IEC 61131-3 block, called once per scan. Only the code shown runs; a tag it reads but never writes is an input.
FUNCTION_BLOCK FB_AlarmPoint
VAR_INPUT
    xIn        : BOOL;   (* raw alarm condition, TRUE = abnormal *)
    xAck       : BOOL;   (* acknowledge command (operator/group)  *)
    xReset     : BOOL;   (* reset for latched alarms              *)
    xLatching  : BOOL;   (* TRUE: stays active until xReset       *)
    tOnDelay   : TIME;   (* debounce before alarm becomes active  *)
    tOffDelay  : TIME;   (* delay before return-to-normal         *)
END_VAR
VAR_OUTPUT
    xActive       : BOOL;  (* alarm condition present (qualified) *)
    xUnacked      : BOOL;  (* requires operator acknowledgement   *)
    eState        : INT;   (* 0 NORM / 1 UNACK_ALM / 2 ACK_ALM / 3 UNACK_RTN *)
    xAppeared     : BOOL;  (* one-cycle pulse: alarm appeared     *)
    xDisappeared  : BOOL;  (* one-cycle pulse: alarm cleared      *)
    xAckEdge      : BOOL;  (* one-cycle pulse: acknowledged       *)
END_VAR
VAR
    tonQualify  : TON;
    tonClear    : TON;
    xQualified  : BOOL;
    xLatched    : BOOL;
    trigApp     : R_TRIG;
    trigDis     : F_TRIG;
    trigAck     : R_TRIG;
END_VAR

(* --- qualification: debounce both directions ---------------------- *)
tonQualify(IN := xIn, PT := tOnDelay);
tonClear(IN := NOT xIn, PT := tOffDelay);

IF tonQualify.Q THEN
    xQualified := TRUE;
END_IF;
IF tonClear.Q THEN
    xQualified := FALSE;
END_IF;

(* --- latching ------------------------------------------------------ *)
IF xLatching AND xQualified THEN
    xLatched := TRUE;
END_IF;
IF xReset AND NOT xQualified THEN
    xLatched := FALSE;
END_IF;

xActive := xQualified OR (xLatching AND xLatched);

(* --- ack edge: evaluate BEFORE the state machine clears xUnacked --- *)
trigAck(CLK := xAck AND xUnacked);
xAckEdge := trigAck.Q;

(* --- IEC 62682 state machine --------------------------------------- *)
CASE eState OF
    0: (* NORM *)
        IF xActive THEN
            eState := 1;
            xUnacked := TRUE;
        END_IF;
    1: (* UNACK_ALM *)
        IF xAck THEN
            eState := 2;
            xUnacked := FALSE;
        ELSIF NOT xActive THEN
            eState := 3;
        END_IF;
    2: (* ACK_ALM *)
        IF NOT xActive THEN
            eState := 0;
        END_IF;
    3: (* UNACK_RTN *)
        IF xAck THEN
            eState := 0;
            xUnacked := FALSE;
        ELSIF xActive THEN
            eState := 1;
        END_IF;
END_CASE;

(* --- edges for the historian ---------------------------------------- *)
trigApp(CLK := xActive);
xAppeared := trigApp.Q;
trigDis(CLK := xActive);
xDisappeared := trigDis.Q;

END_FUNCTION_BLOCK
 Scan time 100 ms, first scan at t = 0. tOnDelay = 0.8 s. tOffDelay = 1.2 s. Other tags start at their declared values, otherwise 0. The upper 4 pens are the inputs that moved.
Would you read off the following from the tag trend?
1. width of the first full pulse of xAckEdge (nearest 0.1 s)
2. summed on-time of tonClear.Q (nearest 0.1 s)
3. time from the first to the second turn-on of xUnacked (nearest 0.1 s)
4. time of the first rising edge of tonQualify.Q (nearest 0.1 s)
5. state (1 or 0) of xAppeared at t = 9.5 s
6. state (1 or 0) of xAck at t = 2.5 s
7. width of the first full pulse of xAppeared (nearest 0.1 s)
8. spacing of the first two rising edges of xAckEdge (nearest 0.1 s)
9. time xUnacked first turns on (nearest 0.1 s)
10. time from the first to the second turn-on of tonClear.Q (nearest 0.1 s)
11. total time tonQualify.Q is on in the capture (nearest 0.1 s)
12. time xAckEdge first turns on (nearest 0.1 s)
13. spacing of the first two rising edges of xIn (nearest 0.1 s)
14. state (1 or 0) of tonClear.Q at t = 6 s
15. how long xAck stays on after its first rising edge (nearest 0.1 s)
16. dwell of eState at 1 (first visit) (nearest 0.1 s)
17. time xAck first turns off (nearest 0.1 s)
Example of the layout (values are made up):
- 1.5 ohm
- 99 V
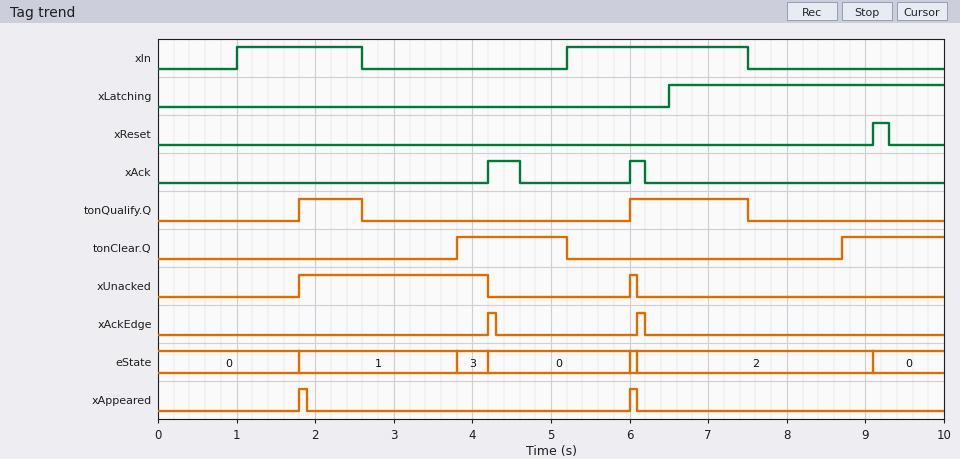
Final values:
- 0.1 s
- 2.7 s
- 4.2 s
- 1.8 s
- 0
- 0
- 0.1 s
- 1.9 s
- 1.8 s
- 4.9 s
- 2.3 s
- 4.2 s
- 4.2 s
- 0
- 0.4 s
- 2.0 s
- 4.6 s
